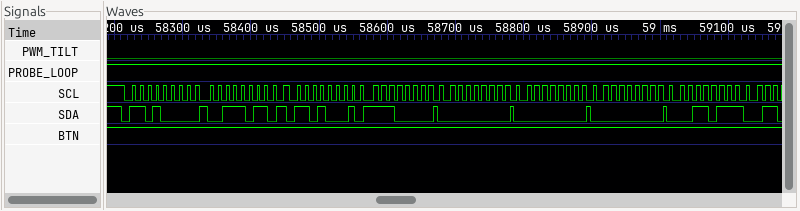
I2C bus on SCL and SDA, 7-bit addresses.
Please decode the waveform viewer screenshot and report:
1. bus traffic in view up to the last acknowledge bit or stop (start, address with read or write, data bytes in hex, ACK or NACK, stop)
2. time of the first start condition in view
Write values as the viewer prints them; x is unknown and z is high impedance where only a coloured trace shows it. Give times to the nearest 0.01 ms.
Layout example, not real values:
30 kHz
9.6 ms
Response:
start, address 68 write ACK, 3B ACK, repeated start, address 68 read ACK, E0 ACK, 00 ACK, 00 ACK, 00 ACK, 37 ACK
58.21 ms
